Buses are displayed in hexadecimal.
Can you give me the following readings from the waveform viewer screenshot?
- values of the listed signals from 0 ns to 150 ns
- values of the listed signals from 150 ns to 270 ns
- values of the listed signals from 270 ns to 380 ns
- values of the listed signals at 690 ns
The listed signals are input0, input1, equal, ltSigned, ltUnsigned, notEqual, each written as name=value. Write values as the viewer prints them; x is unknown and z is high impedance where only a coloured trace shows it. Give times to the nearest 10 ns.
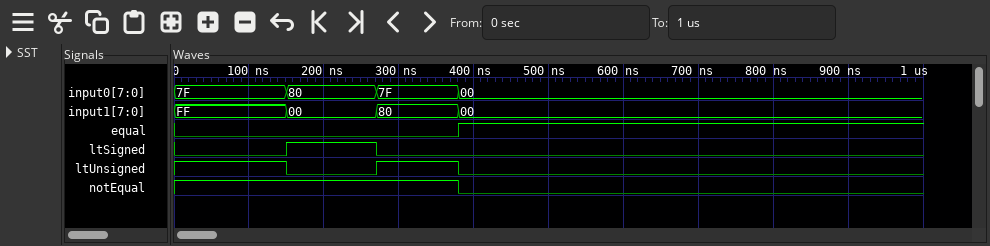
input0=7F, input1=FF, equal=0, ltSigned=0, ltUnsigned=1, notEqual=1
input0=80, input1=00, equal=0, ltSigned=1, ltUnsigned=0, notEqual=1
input0=7F, input1=80, equal=0, ltSigned=0, ltUnsigned=1, notEqual=1
input0=00, input1=00, equal=1, ltSigned=0, ltUnsigned=0, notEqual=0
